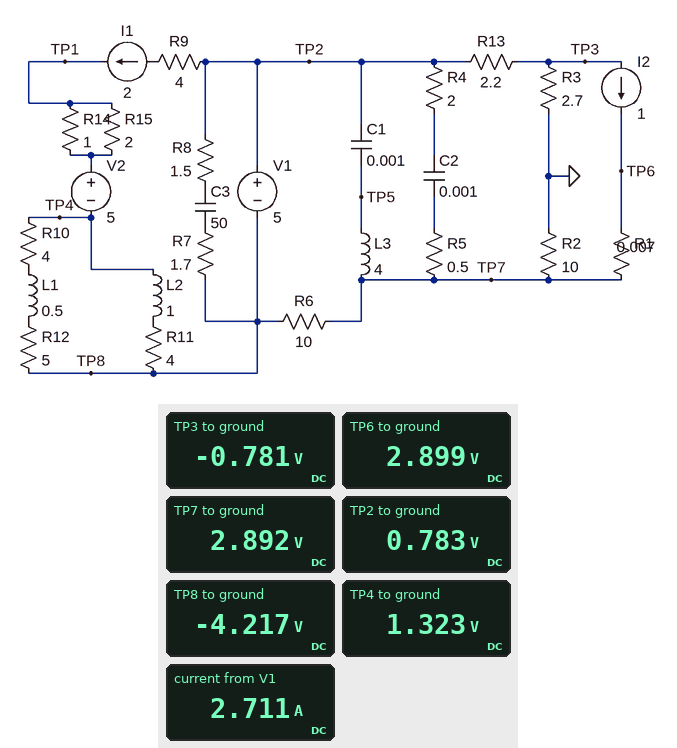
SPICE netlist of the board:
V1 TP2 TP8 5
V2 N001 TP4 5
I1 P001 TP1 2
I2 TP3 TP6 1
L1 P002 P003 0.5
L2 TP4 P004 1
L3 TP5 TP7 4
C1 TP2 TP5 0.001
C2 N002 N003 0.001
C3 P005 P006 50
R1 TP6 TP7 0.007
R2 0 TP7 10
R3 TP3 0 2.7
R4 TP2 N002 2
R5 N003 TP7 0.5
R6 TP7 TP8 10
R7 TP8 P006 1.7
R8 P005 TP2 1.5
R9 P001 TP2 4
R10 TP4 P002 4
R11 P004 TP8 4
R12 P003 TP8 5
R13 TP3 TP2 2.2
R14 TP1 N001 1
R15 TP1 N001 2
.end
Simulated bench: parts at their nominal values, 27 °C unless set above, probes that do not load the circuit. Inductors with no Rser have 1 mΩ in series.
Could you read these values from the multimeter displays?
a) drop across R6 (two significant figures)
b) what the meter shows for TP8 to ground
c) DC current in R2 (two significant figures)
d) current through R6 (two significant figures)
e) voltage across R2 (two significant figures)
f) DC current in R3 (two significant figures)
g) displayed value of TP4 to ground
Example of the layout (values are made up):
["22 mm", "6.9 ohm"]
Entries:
["7.1 V", "-4.217 V", "290 mA", "710 mA", "2.9 V", "290 mA", "1.323 V"]
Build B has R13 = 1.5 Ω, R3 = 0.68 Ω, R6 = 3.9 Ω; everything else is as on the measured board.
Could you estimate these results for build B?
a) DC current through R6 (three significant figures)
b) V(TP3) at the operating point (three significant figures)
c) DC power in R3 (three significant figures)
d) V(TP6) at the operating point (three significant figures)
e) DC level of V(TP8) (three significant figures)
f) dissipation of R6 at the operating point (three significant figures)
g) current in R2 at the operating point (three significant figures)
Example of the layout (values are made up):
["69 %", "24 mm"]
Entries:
["975 mA", "-16.9 mV", "421 µW", "256 mV", "-3.55 V", "3.71 W", "24.9 mA"]
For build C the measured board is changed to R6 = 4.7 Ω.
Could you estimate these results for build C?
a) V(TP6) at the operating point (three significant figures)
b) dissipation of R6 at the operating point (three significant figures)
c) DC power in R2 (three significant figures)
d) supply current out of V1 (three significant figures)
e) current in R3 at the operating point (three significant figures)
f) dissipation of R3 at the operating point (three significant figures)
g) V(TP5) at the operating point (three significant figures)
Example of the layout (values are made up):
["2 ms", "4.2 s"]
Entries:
["976 mV", "3.83 W", "94.0 mW", "2.90 A", "96.9 mA", "25.4 mW", "969 mV"]
